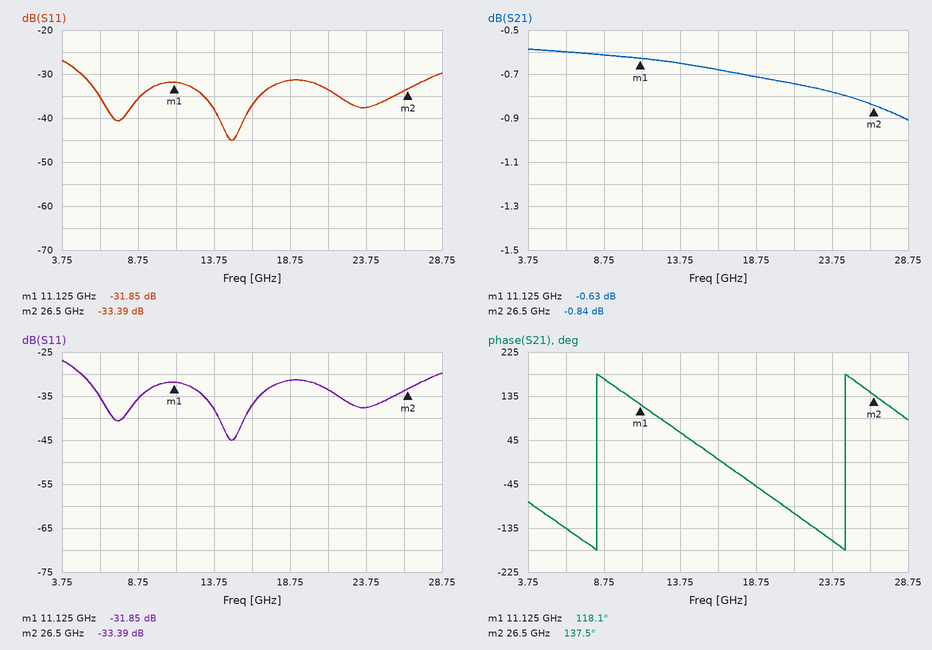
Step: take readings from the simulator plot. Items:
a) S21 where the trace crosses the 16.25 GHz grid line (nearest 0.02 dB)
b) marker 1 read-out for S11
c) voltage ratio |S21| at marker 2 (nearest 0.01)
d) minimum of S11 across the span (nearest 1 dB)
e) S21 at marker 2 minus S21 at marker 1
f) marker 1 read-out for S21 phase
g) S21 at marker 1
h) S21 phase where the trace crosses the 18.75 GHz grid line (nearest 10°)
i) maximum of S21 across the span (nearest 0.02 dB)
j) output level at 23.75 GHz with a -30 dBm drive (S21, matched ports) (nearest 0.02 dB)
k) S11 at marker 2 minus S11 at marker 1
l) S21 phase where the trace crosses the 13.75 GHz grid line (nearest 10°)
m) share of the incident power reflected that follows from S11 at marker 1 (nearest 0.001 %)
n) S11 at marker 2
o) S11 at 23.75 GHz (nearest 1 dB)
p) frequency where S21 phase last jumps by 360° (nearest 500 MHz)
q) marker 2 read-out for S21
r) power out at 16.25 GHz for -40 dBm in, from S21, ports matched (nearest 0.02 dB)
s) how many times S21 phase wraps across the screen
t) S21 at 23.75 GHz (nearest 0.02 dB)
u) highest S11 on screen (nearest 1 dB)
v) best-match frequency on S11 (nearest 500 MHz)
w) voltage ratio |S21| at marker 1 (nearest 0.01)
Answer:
-0.68 dB
-31.85 dB
0.91
-45 dB
-0.21 dB
118.1°
-0.63 dB
-50°
-0.58 dB
-30.78 dBm
-1.54 dB
60°
0.065 %
-33.39 dB
-38 dB
24.5 GHz
-0.84 dB
-40.68 dBm
2
-0.78 dB
-27 dB
15.0 GHz
0.93
